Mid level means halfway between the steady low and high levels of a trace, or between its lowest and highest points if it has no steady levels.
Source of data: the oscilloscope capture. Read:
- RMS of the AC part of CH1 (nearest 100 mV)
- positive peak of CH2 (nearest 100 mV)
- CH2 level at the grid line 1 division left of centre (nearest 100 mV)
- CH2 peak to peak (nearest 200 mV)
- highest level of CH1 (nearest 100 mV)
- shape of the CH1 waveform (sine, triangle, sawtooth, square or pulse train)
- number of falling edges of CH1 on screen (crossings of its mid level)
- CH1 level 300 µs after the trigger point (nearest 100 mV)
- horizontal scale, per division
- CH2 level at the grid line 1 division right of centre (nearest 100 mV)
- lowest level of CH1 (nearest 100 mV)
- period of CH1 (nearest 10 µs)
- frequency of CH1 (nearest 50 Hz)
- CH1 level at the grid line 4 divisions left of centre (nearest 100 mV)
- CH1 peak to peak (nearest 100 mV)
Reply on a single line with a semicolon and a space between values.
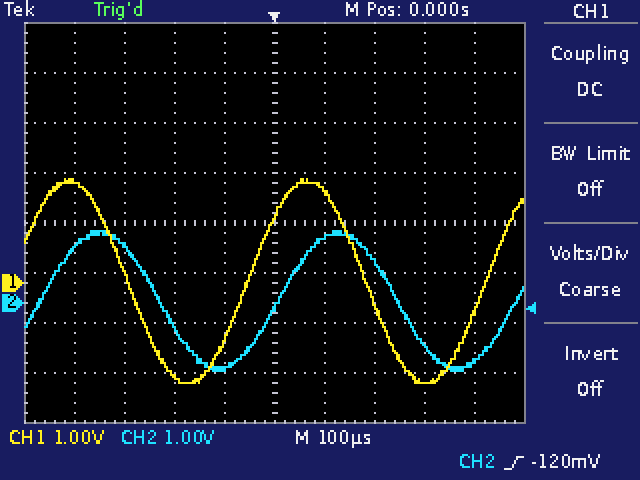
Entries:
1.4 V; 1.4 V; -1.3 V; 2.8 V; 2.1 V; sine; 2; -2.0 V; 100 µs; 1.3 V; -2.0 V; 480 µs; 2.10 kHz; 2.0 V; 4.1 V
